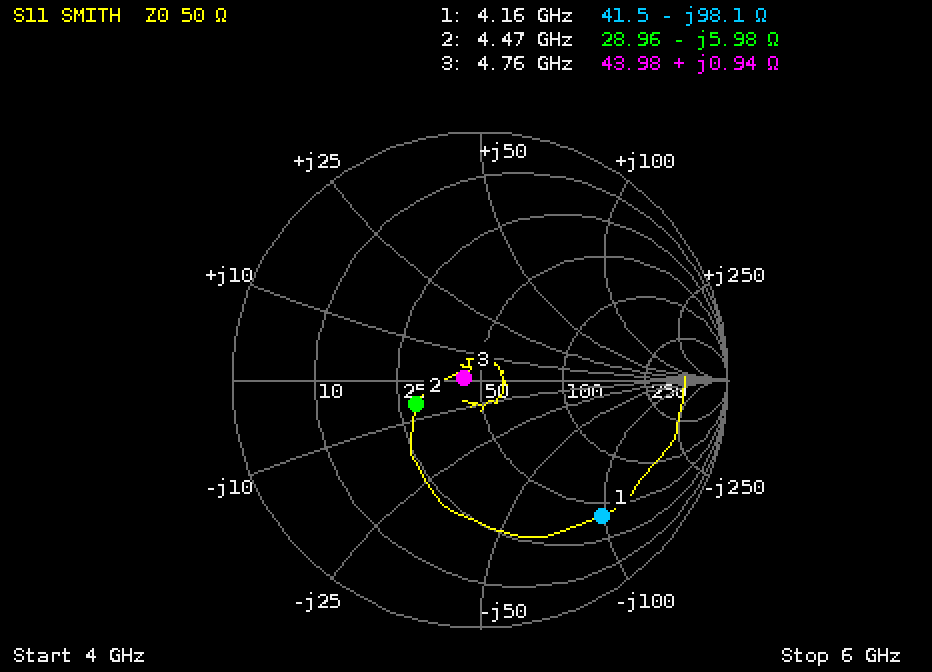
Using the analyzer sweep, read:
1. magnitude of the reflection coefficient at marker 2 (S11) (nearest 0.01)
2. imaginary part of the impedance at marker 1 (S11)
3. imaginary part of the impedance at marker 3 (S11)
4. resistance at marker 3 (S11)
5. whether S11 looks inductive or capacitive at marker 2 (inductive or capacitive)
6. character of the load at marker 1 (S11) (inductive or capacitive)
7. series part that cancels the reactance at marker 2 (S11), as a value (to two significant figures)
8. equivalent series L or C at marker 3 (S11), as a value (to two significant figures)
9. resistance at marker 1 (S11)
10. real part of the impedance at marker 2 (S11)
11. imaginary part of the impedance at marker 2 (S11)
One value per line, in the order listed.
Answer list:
0.28
-98.1 Ω
+0.94 Ω
43.98 Ω
capacitive
capacitive
210 pH
31 pH
41.5 Ω
28.96 Ω
-5.98 Ω
